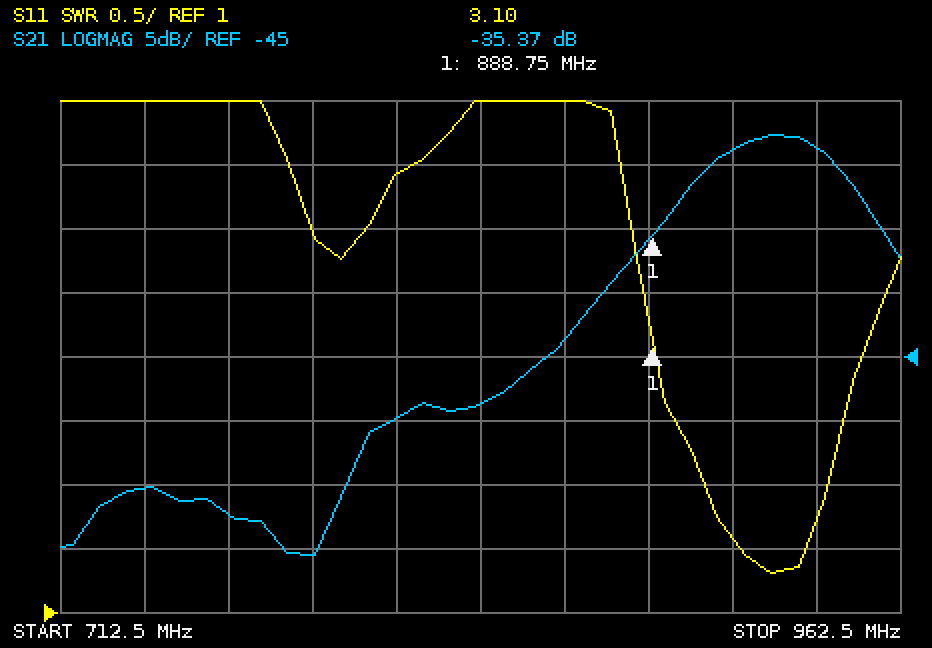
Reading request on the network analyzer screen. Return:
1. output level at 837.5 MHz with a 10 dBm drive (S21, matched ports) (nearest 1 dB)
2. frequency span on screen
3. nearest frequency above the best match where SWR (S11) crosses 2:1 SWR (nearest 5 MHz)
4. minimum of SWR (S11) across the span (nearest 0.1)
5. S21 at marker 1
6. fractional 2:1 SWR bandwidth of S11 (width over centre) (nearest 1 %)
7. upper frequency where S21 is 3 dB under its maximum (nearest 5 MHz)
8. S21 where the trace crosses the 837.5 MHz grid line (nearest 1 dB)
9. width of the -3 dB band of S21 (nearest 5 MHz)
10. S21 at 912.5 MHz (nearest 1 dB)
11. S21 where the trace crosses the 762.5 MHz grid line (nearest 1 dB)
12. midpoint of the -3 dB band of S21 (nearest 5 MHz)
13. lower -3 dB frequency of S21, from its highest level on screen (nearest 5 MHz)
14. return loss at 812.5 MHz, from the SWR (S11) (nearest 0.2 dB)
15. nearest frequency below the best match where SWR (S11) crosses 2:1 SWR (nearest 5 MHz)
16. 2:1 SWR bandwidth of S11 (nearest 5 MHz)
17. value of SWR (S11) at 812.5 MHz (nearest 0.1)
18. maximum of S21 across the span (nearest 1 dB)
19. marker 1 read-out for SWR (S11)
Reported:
-39 dBm
250 MHz
940 MHz
1.3
-35.37 dB
4 %
945 MHz
-49 dB
40 MHz
-29 dB
-57 dB
925 MHz
905 MHz
4.0 dB
905 MHz
35 MHz
4.4
-28 dB
3.10
